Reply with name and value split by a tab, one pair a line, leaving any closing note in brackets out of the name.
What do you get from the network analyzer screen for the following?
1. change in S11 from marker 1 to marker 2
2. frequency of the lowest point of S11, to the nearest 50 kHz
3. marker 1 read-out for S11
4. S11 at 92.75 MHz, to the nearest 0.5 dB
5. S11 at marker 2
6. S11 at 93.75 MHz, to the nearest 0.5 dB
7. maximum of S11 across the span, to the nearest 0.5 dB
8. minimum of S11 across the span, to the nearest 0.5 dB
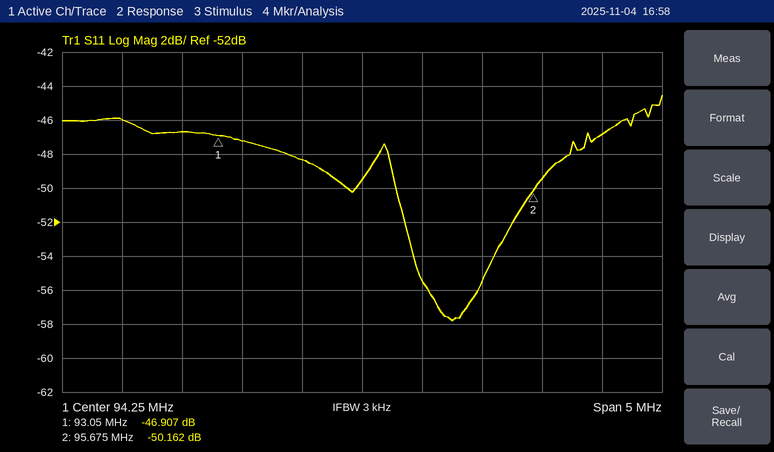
change in S11 from marker 1 to marker 2	-3.255 dB
frequency of the lowest point of S11, to the nearest 50 kHz	95.00 MHz
marker 1 read-out for S11	-46.907 dB
S11 at 92.75 MHz, to the nearest 0.5 dB	-46.5 dB
S11 at marker 2	-50.162 dB
S11 at 93.75 MHz, to the nearest 0.5 dB	-48.5 dB
maximum of S11 across the span, to the nearest 0.5 dB	-44.5 dB
minimum of S11 across the span, to the nearest 0.5 dB	-58.0 dB
